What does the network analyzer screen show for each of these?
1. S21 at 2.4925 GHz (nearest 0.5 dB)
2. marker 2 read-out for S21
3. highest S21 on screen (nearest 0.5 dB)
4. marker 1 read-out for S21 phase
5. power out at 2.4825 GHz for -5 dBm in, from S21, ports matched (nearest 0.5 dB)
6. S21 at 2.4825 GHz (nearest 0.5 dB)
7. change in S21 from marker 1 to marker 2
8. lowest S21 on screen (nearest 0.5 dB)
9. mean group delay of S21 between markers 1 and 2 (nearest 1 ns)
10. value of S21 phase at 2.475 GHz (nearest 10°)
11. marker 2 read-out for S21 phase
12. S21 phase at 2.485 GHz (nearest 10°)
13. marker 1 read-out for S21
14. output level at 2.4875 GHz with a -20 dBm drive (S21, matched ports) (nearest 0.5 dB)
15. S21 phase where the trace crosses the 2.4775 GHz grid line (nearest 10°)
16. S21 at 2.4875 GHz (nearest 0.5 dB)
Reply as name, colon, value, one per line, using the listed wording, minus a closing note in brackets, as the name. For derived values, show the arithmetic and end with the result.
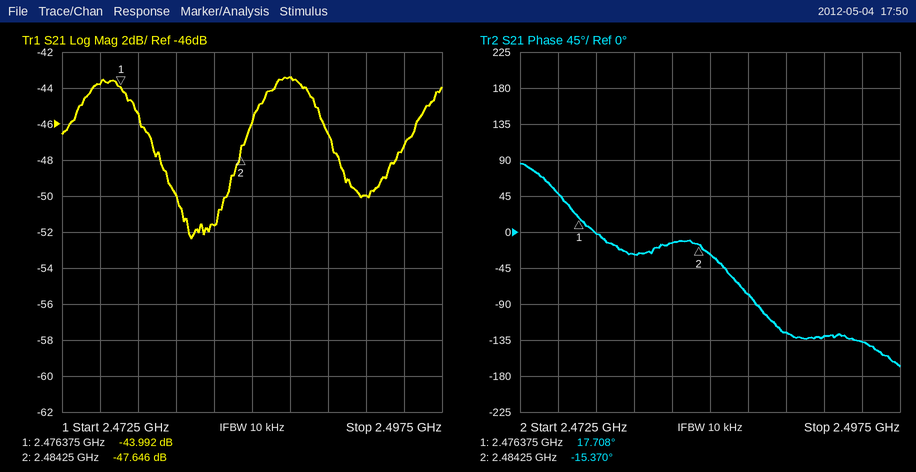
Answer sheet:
S21 at 2.4925 GHz: -50.0 dB
marker 2 read-out for S21: -47.646 dB
highest S21 on screen: -43.5 dB
marker 1 read-out for S21 phase: 17.708°
power out at 2.4825 GHz for -5 dBm in, from S21, ports matched: -5 dBm + (-51.5 dB) = -56.5 dBm
S21 at 2.4825 GHz: -51.5 dB
change in S21 from marker 1 to marker 2: -47.646 − (-43.992) = -3.654 dB
lowest S21 on screen: -52.5 dB
mean group delay of S21 between markers 1 and 2: −(-15.37° − (17.708°))/(360° × 7.875 MHz) ≈ 12 ns
value of S21 phase at 2.475 GHz: 50°
marker 2 read-out for S21 phase: -15.370°
S21 phase at 2.485 GHz: -30°
marker 1 read-out for S21: -43.992 dB
output level at 2.4875 GHz with a -20 dBm drive (S21, matched ports): -20 dBm + (-43.5 dB) = -63.5 dBm
S21 phase where the trace crosses the 2.4775 GHz grid line: 0°
S21 at 2.4875 GHz: -43.5 dB
